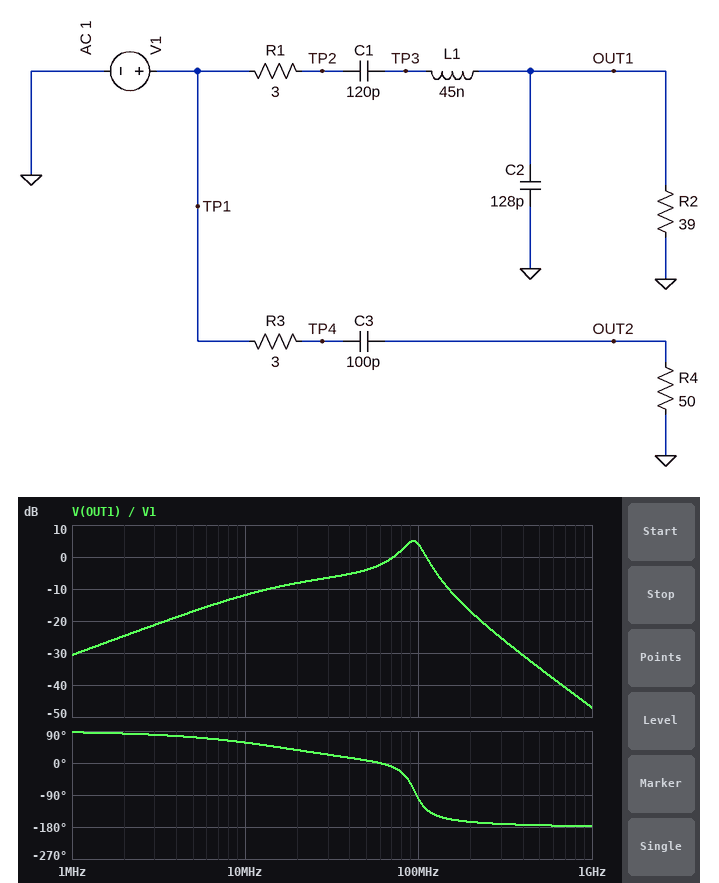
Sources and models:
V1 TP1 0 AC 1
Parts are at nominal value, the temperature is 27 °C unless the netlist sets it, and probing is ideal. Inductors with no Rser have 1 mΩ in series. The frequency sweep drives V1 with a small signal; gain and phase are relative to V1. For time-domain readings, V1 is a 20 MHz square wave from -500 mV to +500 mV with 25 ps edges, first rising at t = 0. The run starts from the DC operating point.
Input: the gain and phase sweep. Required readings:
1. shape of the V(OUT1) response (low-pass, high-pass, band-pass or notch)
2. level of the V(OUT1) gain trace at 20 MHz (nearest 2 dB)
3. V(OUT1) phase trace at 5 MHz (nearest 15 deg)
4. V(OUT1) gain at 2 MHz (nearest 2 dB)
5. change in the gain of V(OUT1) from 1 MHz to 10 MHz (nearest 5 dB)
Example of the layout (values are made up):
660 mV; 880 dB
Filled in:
band-pass; -8 dB; 75 deg; -24 dB; 20 dB
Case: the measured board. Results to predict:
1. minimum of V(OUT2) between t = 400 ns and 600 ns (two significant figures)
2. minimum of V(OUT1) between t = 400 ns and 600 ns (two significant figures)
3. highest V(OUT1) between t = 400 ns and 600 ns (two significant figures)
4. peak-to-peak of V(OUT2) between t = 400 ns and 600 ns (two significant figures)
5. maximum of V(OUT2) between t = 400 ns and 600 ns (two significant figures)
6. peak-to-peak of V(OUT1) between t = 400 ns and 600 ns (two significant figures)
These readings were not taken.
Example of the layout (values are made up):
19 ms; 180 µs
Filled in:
-930 mV; -620 mV; 620 mV; 1.9 V; 930 mV; 1.2 V
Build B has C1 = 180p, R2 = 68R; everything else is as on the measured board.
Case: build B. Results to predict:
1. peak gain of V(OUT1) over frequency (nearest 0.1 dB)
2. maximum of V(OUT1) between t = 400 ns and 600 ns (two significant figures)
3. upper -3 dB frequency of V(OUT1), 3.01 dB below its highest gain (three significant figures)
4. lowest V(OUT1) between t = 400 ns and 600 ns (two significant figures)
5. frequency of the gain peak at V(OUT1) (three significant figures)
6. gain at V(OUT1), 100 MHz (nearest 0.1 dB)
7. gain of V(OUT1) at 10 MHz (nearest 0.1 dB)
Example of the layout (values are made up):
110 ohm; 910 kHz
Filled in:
7.5 dB; 700 mV; 95.8 MHz; -700 mV; 85.6 MHz; 2.6 dB; -6.6 dB
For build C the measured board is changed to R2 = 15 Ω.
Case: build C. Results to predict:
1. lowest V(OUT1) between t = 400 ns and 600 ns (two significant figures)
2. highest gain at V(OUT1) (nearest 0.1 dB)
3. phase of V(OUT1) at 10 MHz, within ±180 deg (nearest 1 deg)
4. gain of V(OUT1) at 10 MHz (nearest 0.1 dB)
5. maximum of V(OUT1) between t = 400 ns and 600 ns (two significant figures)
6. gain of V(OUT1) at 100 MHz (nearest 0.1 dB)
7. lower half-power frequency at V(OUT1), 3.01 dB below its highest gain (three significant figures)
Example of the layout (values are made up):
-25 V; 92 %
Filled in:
-410 mV; 0.1 dB; 75 deg; -19.0 dB; 410 mV; -1.9 dB; 62.0 MHz
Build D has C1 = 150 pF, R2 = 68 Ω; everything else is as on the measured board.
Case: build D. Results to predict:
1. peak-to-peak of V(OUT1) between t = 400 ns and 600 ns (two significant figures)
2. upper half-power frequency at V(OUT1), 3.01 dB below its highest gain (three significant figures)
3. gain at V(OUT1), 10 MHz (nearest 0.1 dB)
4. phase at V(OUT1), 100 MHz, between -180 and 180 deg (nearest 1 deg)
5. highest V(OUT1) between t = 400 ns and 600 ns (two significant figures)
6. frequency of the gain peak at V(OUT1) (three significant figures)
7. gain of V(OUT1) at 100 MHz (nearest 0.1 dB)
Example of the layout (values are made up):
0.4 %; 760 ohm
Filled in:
1.4 V; 99.0 MHz; -7.6 dB; -127 deg; 680 mV; 89.2 MHz; 4.1 dB
